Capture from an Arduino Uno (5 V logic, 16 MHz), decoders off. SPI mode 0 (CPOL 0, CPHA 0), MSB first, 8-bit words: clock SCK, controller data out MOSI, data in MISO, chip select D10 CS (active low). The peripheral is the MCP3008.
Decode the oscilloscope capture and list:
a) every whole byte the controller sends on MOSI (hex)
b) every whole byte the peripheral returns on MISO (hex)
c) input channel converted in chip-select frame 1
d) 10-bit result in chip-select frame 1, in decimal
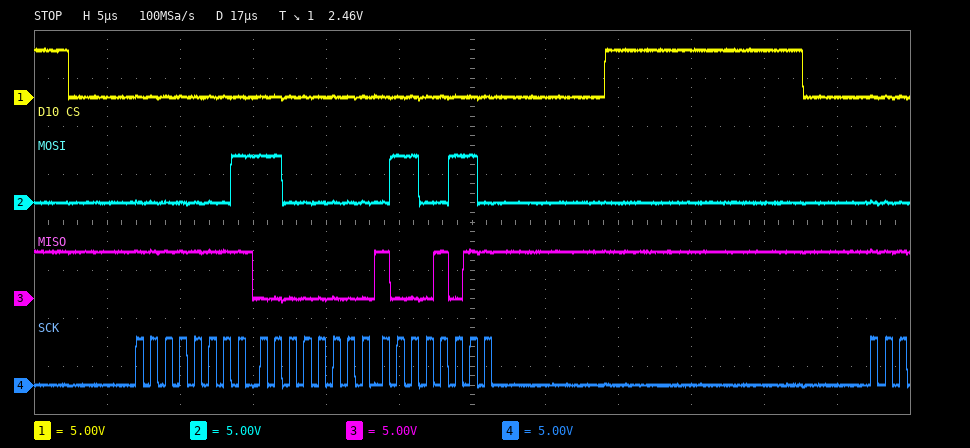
01 C0 66
FF 00 8B
4
139
